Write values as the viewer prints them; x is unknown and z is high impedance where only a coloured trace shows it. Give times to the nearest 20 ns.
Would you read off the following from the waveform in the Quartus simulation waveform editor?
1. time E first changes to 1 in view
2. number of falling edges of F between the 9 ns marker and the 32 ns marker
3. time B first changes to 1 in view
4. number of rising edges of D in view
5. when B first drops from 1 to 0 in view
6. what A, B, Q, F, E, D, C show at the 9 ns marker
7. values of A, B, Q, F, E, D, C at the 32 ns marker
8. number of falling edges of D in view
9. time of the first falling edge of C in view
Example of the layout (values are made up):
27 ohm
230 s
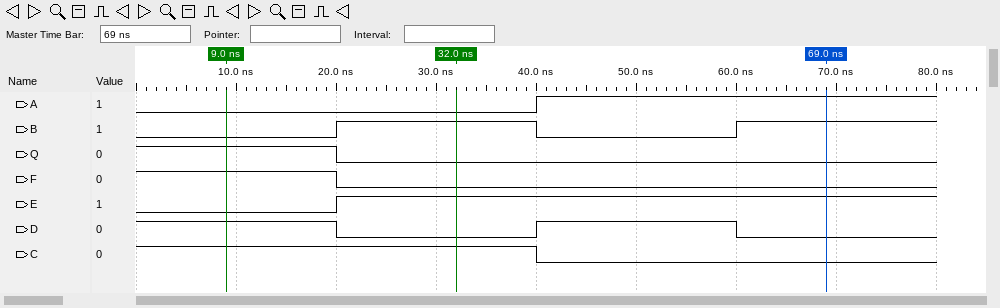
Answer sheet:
20 ns
1
20 ns
1
40 ns
A=0, B=0, Q=1, F=1, E=0, D=1, C=1
A=0, B=1, Q=0, F=0, E=1, D=0, C=1
2
40 ns
